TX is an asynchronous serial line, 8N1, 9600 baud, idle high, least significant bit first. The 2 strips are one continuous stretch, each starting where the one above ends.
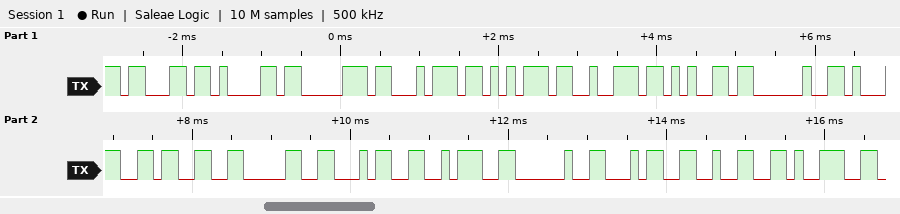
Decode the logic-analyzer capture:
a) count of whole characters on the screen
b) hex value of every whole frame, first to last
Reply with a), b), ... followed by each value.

a) 17
b) 0x63 0x61 0x70 0x74 0x75 0x72 0x65 0x20 0x31 0x33 0x30 0x34 0x3A 0x20 0x34 0x32 0x39
